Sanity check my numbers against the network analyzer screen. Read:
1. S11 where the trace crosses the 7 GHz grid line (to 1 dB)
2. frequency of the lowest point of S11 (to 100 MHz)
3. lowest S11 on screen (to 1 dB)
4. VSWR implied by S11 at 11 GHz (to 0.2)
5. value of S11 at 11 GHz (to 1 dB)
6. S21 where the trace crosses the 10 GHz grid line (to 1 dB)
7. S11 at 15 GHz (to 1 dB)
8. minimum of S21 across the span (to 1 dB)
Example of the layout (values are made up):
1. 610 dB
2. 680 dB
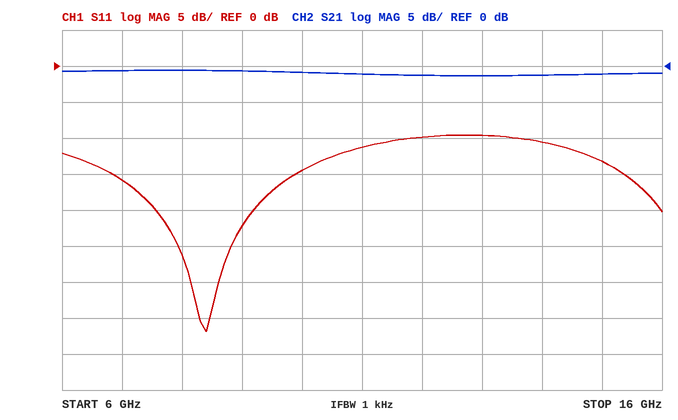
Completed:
1. -16 dB
2. 8.4 GHz
3. -37 dB
4. 1.8
5. -11 dB
6. -1 dB
7. -13 dB
8. -1 dB
